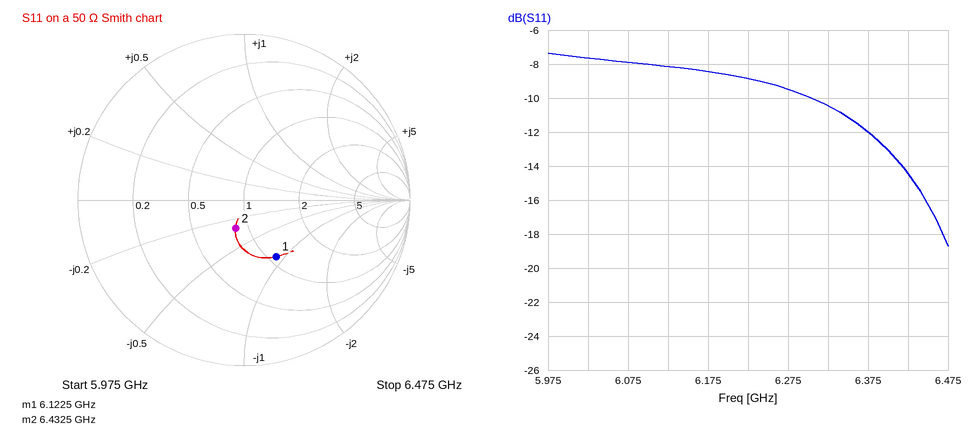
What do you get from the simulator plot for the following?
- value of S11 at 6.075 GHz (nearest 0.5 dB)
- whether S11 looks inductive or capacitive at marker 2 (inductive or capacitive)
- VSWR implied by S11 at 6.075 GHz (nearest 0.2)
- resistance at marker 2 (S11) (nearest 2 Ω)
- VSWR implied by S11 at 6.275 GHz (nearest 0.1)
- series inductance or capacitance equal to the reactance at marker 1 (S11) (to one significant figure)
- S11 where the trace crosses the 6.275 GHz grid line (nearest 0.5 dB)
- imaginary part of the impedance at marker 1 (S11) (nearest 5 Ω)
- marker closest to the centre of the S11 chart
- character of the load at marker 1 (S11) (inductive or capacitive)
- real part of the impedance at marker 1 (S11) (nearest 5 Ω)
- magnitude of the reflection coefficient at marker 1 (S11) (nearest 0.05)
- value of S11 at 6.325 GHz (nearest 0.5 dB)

-8.0 dB
capacitive
2.4
42 Ω
2.0
600 fF
-9.5 dB
-45 Ω
marker 2
capacitive
55 Ω
0.40
-10.5 dB
